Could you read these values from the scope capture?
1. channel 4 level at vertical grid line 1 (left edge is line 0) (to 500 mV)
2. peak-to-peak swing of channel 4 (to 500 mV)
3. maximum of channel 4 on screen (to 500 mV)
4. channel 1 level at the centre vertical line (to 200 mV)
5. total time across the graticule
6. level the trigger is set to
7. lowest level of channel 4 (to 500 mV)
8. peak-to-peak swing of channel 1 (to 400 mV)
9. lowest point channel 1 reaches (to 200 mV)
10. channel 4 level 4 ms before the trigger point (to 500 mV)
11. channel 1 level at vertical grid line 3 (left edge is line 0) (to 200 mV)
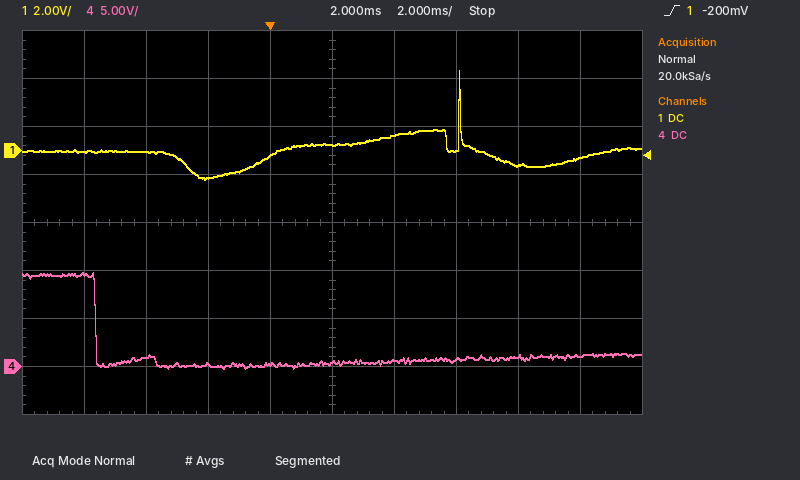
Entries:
9.5 V
10.0 V
10.0 V
200 mV
20 ms
-200 mV
0.0 V
4.4 V
-1.2 V
1.0 V
-1.2 V
